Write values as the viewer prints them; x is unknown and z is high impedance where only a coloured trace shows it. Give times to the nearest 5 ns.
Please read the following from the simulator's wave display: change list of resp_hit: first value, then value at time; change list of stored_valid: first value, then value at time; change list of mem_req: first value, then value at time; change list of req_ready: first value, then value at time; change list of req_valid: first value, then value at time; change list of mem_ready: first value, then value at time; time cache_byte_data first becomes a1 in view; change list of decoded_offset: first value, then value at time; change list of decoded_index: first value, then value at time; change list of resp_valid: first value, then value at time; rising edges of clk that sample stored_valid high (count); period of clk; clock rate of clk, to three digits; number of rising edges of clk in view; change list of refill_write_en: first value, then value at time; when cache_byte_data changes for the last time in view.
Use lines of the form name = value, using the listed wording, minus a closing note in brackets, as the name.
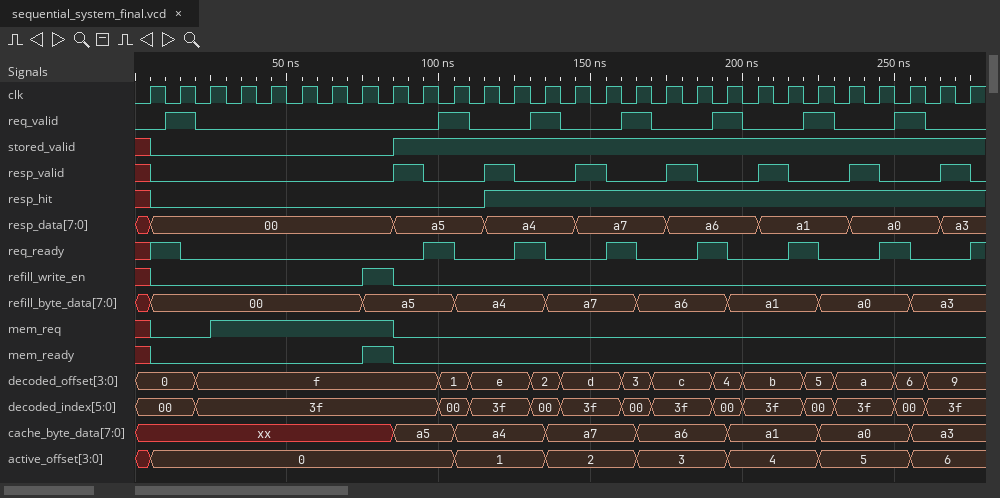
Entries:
change list of resp_hit: first value, then value at time = x, 0 at 5 ns, 1 at 115 ns
change list of stored_valid: first value, then value at time = x, 0 at 5 ns, 1 at 85 ns
change list of mem_req: first value, then value at time = x, 0 at 5 ns, 1 at 25 ns, 0 at 85 ns
change list of req_ready: first value, then value at time = x, 1 at 5 ns, 0 at 15 ns, 1 at 95 ns, 0 at 105 ns, 1 at 125 ns, 0 at 135 ns, 1 at 155 ns, 0 at 165 ns, 1 at 185 ns, 0 at 195 ns, 1 at 215 ns, 0 at 225 ns, 1 at 245 ns, 0 at 255 ns, 1 at 275 ns
change list of req_valid: first value, then value at time = 0, 1 at 10 ns, 0 at 20 ns, 1 at 100 ns, 0 at 110 ns, 1 at 130 ns, 0 at 140 ns, 1 at 160 ns, 0 at 170 ns, 1 at 190 ns, 0 at 200 ns, 1 at 220 ns, 0 at 230 ns, 1 at 250 ns, 0 at 260 ns
change list of mem_ready: first value, then value at time = x, 0 at 5 ns, 1 at 75 ns, 0 at 85 ns
time cache_byte_data first becomes a1 in view = 195 ns
change list of decoded_offset: first value, then value at time = 0, f at 20 ns, 1 at 100 ns, e at 110 ns, 2 at 130 ns, d at 140 ns, 3 at 160 ns, c at 170 ns, 4 at 190 ns, b at 200 ns, 5 at 220 ns, a at 230 ns, 6 at 250 ns, 9 at 260 ns
change list of decoded_index: first value, then value at time = 00, 3f at 20 ns, 00 at 100 ns, 3f at 110 ns, 00 at 130 ns, 3f at 140 ns, 00 at 160 ns, 3f at 170 ns, 00 at 190 ns, 3f at 200 ns, 00 at 220 ns, 3f at 230 ns, 00 at 250 ns, 3f at 260 ns
change list of resp_valid: first value, then value at time = x, 0 at 5 ns, 1 at 85 ns, 0 at 95 ns, 1 at 115 ns, 0 at 125 ns, 1 at 145 ns, 0 at 155 ns, 1 at 175 ns, 0 at 185 ns, 1 at 205 ns, 0 at 215 ns, 1 at 235 ns, 0 at 245 ns, 1 at 265 ns, 0 at 275 ns
rising edges of clk that sample stored_valid high = 19
period of clk = 10 ns
clock rate of clk, to three digits = 100 MHz
number of rising edges of clk in view = 28
change list of refill_write_en: first value, then value at time = x, 0 at 5 ns, 1 at 75 ns, 0 at 85 ns
when cache_byte_data changes for the last time in view = 255 ns
